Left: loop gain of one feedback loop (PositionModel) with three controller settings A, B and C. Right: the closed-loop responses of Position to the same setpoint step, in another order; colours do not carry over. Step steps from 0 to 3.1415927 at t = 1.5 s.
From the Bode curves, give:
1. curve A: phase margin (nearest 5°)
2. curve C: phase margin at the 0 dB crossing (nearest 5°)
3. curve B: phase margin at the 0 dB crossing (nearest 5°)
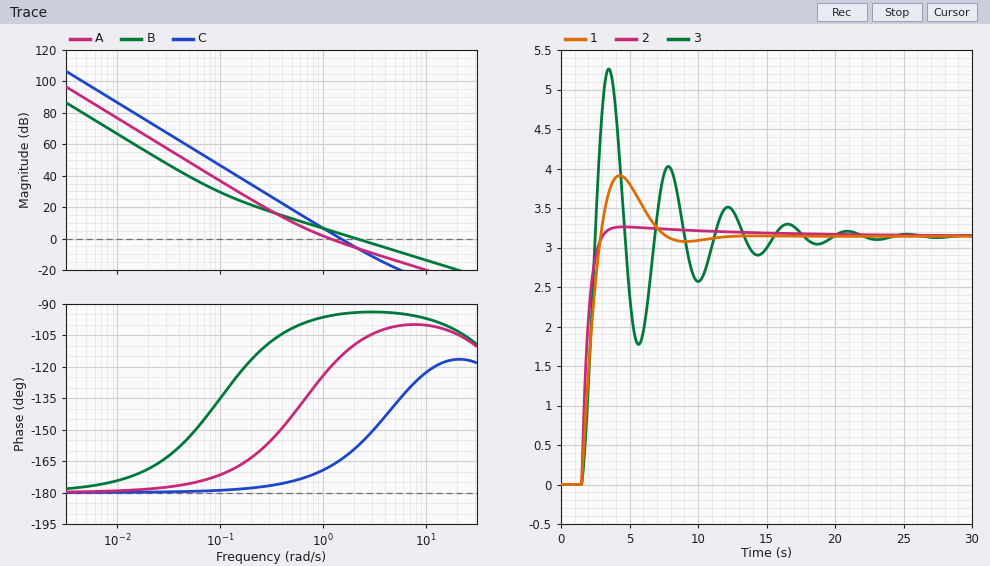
60°
15°
85°
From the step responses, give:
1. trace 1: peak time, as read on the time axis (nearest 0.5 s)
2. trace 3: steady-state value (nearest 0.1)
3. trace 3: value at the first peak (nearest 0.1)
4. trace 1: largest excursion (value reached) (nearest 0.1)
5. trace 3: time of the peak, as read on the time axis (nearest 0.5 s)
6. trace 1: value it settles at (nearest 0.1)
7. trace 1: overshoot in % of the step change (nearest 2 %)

4.5 s
3.1
5.3
3.9
3.5 s
3.1
24 %
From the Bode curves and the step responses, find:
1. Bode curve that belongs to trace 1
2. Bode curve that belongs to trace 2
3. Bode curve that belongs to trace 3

A
B
C
